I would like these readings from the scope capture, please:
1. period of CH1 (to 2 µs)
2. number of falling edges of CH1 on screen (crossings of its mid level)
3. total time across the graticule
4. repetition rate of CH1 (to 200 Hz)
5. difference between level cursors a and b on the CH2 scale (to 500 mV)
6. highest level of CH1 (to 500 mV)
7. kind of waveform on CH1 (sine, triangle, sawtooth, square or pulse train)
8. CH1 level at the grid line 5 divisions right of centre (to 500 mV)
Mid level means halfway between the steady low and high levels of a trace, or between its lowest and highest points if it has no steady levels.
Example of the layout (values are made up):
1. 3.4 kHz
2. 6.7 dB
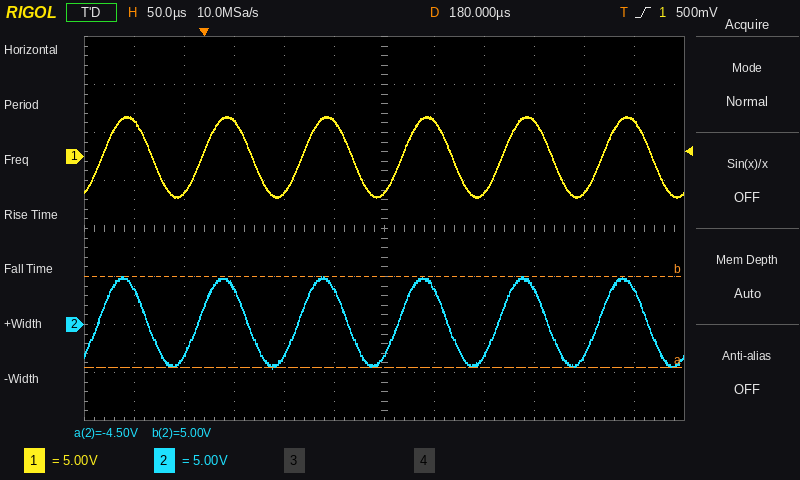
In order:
1. 100 µs
2. 6
3. 600 µs
4. 10.0 kHz
5. 9.5 V
6. 4.0 V
7. sine
8. 3.5 V
